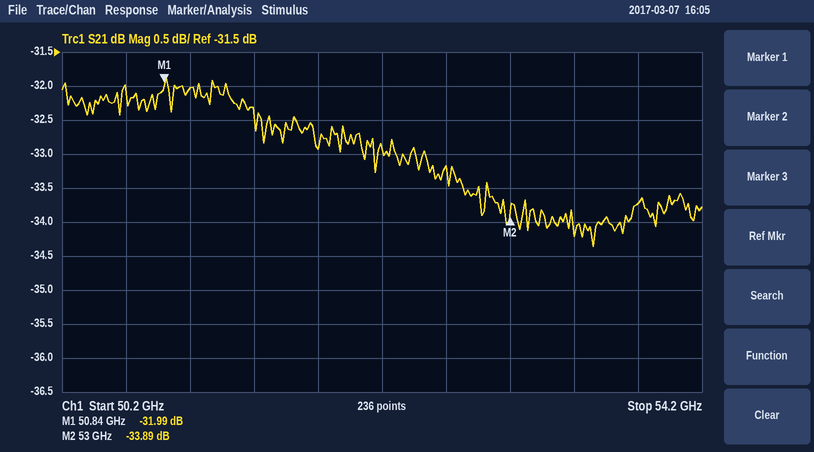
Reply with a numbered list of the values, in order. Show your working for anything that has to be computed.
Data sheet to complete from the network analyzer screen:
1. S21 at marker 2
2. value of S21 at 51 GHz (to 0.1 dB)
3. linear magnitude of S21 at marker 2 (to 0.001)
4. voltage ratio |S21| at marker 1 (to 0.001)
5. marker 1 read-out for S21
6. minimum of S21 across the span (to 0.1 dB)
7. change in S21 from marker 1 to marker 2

1. -33.89 dB
2. -32.0 dB
3. 10^(-33.89/20) ≈ 0.020
4. 10^(-31.99/20) ≈ 0.025
5. -31.99 dB
6. -34.4 dB
7. -33.89 − (-31.99) = -1.90 dB
